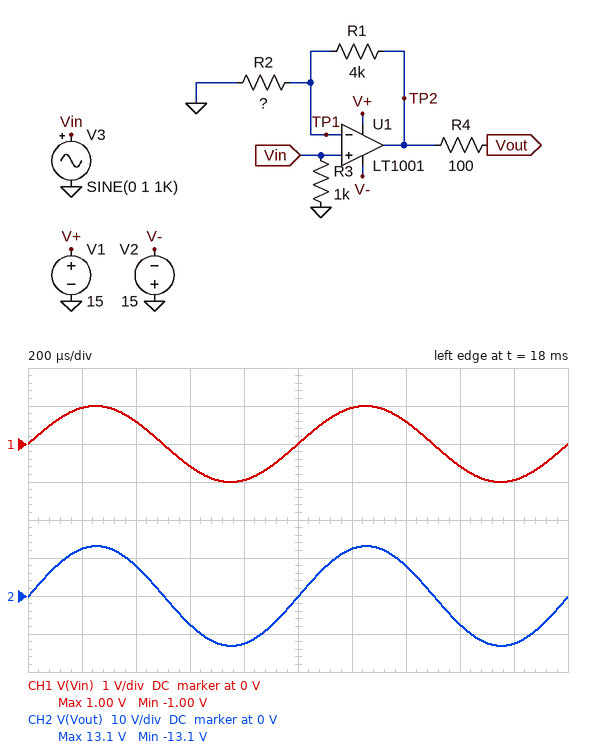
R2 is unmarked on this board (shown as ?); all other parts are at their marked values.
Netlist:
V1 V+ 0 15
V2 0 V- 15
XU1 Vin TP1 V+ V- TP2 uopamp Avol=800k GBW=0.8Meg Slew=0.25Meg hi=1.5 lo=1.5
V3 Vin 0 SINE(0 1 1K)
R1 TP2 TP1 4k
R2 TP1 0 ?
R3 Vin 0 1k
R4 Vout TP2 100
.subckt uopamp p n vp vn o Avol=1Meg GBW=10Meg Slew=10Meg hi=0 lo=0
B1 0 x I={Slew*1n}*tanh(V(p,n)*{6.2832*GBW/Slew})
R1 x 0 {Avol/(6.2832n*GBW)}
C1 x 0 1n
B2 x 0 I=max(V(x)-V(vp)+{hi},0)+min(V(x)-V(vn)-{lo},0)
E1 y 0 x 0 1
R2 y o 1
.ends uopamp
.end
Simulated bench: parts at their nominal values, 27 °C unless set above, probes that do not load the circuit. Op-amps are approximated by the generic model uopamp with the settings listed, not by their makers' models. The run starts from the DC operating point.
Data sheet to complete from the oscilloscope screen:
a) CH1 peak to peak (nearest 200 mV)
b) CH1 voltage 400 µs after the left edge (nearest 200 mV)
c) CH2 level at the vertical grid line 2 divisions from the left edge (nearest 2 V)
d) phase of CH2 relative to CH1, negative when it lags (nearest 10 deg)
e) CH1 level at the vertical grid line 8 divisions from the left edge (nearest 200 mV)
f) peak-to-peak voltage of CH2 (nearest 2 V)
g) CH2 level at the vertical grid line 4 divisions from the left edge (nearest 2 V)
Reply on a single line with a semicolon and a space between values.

2.0 V; 600 mV; 8 V; 0 deg; -600 mV; 26 V; -12 V
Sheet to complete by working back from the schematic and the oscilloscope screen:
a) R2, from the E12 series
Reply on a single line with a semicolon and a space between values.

330 Ω
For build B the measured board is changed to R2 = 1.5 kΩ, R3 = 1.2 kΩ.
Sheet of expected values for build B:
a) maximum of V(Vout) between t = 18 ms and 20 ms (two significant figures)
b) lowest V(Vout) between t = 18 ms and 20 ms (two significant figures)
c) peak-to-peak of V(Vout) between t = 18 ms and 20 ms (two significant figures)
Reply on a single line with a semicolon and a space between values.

3.7 V; -3.7 V; 7.3 V
